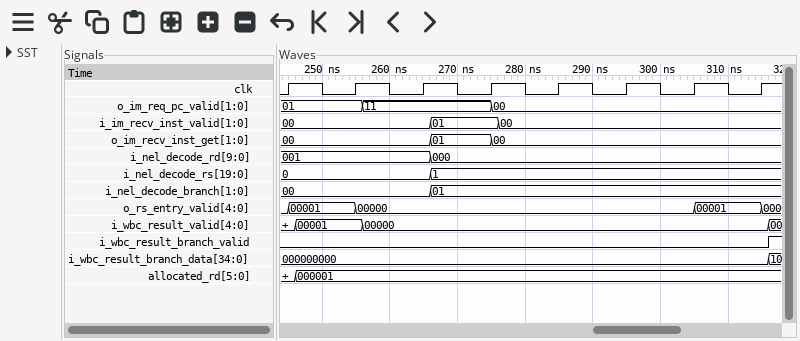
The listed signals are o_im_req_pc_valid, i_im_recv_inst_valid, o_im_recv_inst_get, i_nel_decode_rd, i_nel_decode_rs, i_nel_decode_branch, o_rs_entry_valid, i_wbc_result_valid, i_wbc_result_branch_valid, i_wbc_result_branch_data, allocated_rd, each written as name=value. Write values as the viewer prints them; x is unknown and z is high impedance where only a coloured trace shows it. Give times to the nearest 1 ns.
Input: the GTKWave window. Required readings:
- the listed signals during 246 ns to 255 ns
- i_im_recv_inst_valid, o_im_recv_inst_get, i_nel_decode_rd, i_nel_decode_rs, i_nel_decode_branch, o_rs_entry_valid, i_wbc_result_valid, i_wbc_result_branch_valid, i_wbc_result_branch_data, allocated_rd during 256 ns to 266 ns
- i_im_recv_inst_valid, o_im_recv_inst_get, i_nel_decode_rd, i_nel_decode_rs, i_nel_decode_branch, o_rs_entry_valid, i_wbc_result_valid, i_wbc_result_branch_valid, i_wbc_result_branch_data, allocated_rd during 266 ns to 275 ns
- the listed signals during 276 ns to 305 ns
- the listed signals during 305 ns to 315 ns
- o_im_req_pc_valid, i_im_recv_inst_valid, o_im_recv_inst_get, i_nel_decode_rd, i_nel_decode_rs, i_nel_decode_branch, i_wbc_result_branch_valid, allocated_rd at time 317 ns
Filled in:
o_im_req_pc_valid=01, i_im_recv_inst_valid=00, o_im_recv_inst_get=00, i_nel_decode_rd=001, i_nel_decode_rs=0, i_nel_decode_branch=00, o_rs_entry_valid=00001, i_wbc_result_valid=00001, i_wbc_result_branch_valid=0, i_wbc_result_branch_data=000000000, allocated_rd=000001
i_im_recv_inst_valid=00, o_im_recv_inst_get=00, i_nel_decode_rd=001, i_nel_decode_rs=0, i_nel_decode_branch=00, o_rs_entry_valid=00000, i_wbc_result_valid=00000, i_wbc_result_branch_valid=0, i_wbc_result_branch_data=000000000, allocated_rd=000001
i_im_recv_inst_valid=01, o_im_recv_inst_get=01, i_nel_decode_rd=000, i_nel_decode_rs=1, i_nel_decode_branch=01, o_rs_entry_valid=00000, i_wbc_result_valid=00000, i_wbc_result_branch_valid=0, i_wbc_result_branch_data=000000000, allocated_rd=000001
o_im_req_pc_valid=00, i_im_recv_inst_valid=00, o_im_recv_inst_get=00, i_nel_decode_rd=000, i_nel_decode_rs=1, i_nel_decode_branch=01, o_rs_entry_valid=00000, i_wbc_result_valid=00000, i_wbc_result_branch_valid=0, i_wbc_result_branch_data=000000000, allocated_rd=000001
o_im_req_pc_valid=00, i_im_recv_inst_valid=00, o_im_recv_inst_get=00, i_nel_decode_rd=000, i_nel_decode_rs=1, i_nel_decode_branch=01, o_rs_entry_valid=00001, i_wbc_result_valid=00000, i_wbc_result_branch_valid=0, i_wbc_result_branch_data=000000000, allocated_rd=000001
o_im_req_pc_valid=00, i_im_recv_inst_valid=00, o_im_recv_inst_get=00, i_nel_decode_rd=000, i_nel_decode_rs=1, i_nel_decode_branch=01, i_wbc_result_branch_valid=1, allocated_rd=000001
